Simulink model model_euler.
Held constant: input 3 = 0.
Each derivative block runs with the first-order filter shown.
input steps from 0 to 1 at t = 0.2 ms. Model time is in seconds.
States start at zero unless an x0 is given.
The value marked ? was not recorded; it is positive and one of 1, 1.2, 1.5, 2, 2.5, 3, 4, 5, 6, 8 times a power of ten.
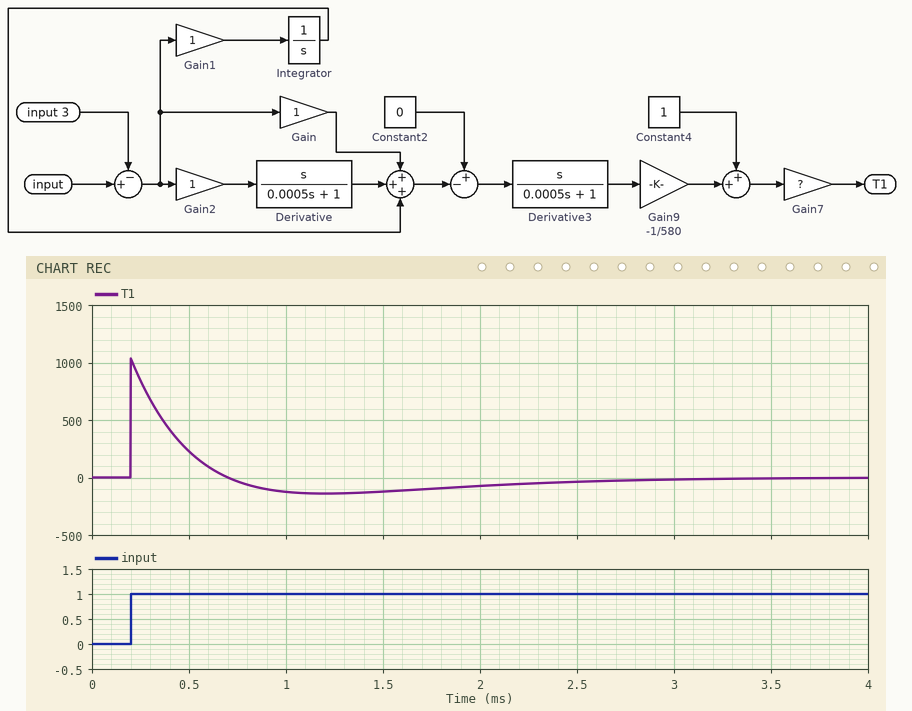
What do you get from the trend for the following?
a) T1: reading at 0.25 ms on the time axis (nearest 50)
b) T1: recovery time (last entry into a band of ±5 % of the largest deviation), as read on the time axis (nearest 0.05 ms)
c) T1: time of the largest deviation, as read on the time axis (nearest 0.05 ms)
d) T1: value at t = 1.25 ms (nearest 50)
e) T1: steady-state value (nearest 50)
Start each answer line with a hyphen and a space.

- 850
- 2.25 ms
- 0.20 ms
- -150
- 0
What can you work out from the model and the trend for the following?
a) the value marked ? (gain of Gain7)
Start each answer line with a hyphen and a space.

- 0.15
